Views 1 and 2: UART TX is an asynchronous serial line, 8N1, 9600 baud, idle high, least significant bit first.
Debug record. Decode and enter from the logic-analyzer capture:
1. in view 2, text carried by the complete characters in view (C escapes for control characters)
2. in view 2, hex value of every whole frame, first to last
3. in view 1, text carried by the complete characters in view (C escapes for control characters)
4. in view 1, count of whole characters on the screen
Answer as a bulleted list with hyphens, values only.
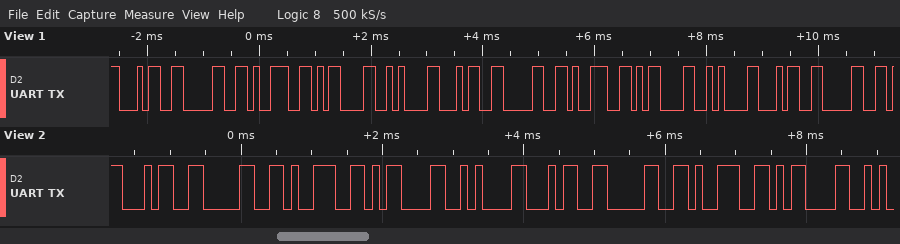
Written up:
- "409\r\n409\r"
- 0x34 0x30 0x39 0x0D 0x0A 0x34 0x30 0x39 0x0D
- "409\r\n409\r\n40"
- 12
